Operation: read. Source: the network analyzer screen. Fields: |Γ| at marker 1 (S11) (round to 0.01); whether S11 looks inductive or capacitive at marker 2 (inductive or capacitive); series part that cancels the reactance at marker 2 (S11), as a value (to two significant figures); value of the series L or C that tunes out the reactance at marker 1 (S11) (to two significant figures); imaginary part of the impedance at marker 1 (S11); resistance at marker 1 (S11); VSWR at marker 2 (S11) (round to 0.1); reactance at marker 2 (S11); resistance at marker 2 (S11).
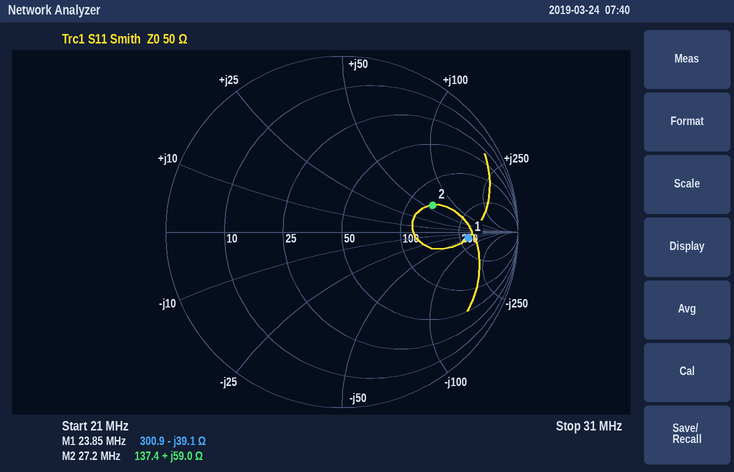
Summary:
0.72
inductive
99 pF
260 nH
-39.1 Ω
300.9 Ω
3.3
+59.0 Ω
137.4 Ω
